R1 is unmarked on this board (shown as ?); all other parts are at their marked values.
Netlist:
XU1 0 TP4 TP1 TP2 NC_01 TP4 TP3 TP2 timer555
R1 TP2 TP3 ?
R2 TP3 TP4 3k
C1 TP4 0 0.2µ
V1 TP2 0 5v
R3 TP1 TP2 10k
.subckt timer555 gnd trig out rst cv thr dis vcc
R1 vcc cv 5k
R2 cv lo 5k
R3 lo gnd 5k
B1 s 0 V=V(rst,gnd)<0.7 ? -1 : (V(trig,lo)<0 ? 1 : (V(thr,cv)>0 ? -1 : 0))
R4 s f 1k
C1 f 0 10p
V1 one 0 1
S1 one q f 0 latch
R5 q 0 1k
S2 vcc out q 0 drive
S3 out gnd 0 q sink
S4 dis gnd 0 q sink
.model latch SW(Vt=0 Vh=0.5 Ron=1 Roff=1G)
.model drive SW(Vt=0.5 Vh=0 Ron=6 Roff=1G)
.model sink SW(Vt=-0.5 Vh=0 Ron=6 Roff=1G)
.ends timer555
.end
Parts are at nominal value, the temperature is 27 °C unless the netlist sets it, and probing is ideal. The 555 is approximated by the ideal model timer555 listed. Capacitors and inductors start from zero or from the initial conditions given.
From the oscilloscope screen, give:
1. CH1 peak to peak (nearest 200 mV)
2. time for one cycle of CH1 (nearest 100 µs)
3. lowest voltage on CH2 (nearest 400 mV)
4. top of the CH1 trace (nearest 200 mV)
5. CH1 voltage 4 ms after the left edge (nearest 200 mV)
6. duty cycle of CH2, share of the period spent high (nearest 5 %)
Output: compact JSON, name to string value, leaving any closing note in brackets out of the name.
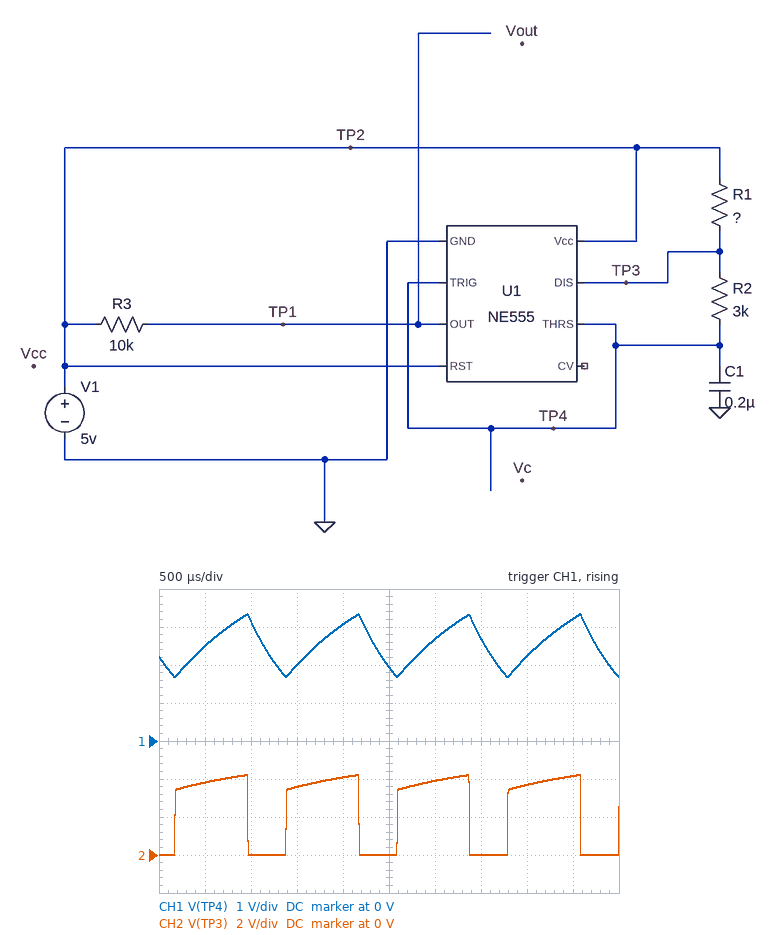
{"CH1 peak to peak": "1.6 V", "time for one cycle of CH1": "1.2 ms", "lowest voltage on CH2": "0 V", "top of the CH1 trace": "3.4 V", "CH1 voltage 4 ms after the left edge": "2.2 V", "duty cycle of CH2, share of the period spent high": "65 %"}
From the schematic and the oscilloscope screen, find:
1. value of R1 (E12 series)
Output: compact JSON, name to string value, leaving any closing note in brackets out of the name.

{"value of R1": "2.7 kΩ"}
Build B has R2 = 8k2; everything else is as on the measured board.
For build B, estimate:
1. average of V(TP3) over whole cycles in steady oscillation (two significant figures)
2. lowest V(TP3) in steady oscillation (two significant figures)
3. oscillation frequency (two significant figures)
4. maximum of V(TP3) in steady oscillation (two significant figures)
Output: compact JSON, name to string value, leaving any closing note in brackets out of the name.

{"average of V(TP3) over whole cycles in steady oscillation": "2.5 V", "lowest V(TP3) in steady oscillation": "12 mV", "oscillation frequency": "380 Hz", "maximum of V(TP3) in steady oscillation": "4.6 V"}
